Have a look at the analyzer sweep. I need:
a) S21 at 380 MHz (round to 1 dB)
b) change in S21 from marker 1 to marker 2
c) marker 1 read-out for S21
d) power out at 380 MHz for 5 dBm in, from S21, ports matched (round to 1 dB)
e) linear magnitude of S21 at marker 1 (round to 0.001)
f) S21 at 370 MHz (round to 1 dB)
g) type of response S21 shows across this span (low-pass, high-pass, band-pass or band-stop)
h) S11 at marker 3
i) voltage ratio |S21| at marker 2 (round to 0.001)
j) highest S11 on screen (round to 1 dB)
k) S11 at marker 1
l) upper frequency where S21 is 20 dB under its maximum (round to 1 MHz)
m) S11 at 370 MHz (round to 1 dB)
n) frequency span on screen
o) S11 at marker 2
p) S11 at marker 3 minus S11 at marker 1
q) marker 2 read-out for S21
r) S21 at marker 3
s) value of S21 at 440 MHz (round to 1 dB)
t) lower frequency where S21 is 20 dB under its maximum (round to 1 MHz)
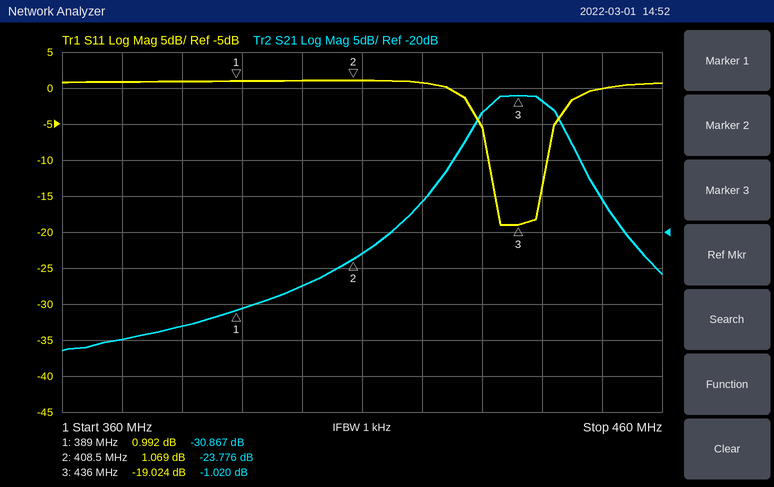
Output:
-33 dB
7.091 dB
-30.867 dB
-28 dBm
0.029
-35 dB
band-pass
-19.024 dB
0.065
1 dB
0.992 dB
455 MHz
1 dB
100 MHz
1.069 dB
-20.016 dB
-23.776 dB
-1.020 dB
-2 dB
413 MHz
